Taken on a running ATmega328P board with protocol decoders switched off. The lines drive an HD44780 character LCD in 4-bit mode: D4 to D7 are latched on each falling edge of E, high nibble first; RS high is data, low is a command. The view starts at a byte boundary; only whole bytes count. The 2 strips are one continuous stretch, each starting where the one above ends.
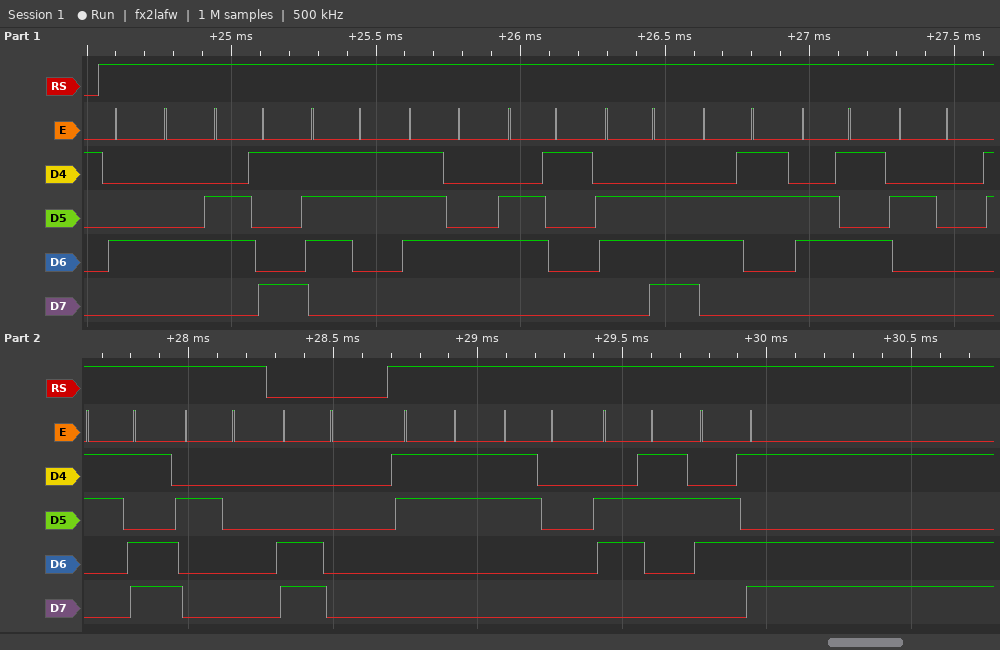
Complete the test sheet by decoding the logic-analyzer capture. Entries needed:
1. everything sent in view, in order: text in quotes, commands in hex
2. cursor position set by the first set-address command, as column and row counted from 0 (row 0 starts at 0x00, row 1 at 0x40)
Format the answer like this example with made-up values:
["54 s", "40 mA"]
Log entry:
["\"Distance = \" 0xC0 \"30cm\"", "column 0, row 1"]
